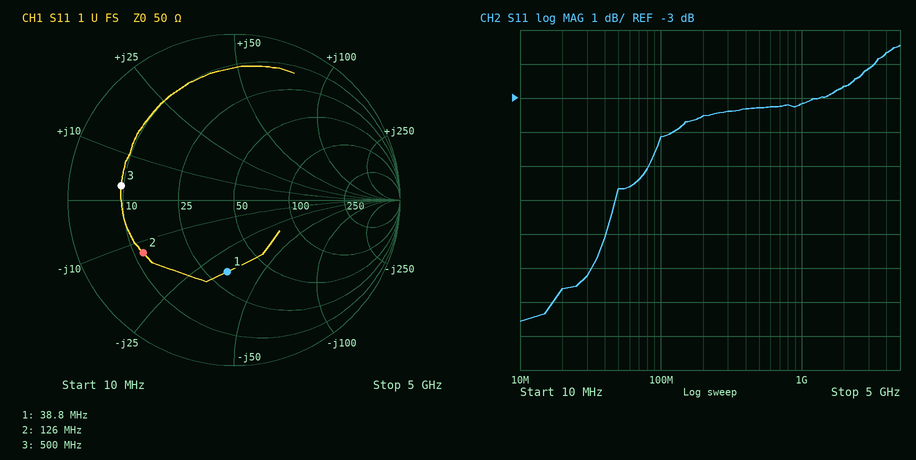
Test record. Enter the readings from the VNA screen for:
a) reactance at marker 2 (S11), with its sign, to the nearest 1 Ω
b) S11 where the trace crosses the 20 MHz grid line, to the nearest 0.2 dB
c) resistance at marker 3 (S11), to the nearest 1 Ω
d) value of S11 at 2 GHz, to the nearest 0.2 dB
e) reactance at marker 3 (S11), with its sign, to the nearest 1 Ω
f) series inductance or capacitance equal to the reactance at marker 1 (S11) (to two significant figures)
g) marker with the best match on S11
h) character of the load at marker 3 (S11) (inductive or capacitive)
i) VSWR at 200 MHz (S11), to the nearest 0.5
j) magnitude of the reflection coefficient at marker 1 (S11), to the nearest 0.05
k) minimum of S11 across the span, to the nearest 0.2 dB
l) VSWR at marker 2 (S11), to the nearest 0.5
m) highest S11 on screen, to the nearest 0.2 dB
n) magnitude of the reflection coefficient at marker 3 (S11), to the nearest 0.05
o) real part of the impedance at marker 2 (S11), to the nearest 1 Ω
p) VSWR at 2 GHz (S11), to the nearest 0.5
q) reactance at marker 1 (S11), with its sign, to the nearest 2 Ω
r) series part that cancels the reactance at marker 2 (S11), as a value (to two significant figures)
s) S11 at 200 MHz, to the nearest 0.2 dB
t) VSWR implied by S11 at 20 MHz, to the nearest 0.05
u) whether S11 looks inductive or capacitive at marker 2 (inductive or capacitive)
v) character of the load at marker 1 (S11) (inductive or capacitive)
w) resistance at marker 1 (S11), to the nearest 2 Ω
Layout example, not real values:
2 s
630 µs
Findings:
-13 Ω
-8.6 dB
9 Ω
-2.6 dB
+3 Ω
120 pF
marker 1
inductive
5.0
0.45
-9.6 dB
4.5
-1.4 dB
0.70
12 Ω
6.5
-34 Ω
16 nH
-3.6 dB
2.20
capacitive
capacitive
32 Ω
